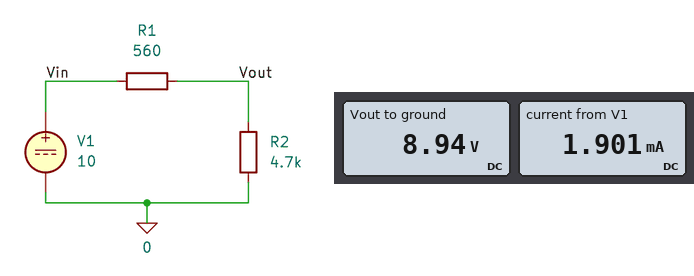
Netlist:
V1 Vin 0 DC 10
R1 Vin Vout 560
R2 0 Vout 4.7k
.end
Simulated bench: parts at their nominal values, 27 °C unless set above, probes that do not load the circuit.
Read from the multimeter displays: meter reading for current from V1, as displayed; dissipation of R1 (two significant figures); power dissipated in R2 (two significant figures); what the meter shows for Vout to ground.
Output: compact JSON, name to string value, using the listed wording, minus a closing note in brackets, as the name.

{"meter reading for current from V1, as displayed": "1.901 mA", "dissipation of R1": "2.0 mW", "power dissipated in R2": "17 mW", "what the meter shows for Vout to ground": "8.94 V"}
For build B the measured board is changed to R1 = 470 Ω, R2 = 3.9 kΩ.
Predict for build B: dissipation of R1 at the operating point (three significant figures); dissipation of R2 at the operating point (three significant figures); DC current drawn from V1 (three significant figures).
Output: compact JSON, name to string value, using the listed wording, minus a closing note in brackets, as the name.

{"dissipation of R1 at the operating point": "2.46 mW", "dissipation of R2 at the operating point": "20.4 mW", "DC current drawn from V1": "2.29 mA"}
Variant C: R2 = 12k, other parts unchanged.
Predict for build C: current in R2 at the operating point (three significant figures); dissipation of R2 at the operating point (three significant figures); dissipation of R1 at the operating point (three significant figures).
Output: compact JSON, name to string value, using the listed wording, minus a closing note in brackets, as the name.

{"current in R2 at the operating point": "796 µA", "dissipation of R2 at the operating point": "7.61 mW", "dissipation of R1 at the operating point": "355 µW"}
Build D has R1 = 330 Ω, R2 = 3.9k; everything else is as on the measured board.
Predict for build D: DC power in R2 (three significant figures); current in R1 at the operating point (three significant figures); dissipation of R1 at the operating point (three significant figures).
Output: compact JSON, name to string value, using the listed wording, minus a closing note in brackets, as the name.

{"DC power in R2": "21.8 mW", "current in R1 at the operating point": "2.36 mA", "dissipation of R1 at the operating point": "1.84 mW"}
